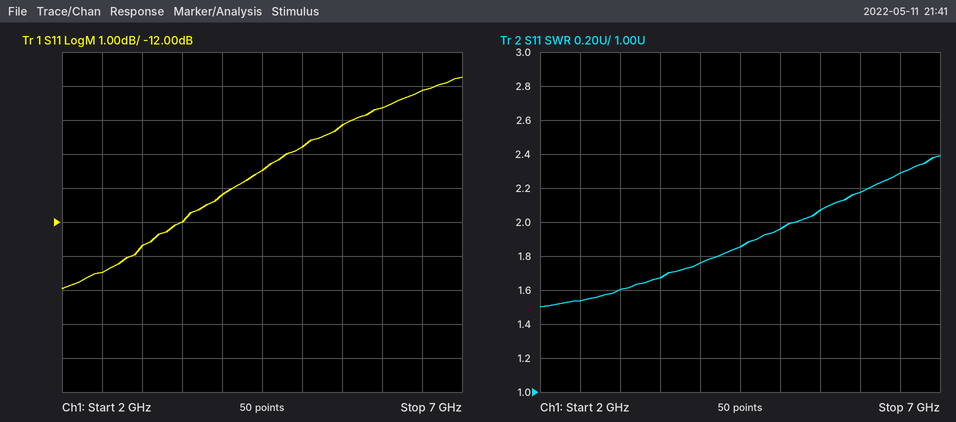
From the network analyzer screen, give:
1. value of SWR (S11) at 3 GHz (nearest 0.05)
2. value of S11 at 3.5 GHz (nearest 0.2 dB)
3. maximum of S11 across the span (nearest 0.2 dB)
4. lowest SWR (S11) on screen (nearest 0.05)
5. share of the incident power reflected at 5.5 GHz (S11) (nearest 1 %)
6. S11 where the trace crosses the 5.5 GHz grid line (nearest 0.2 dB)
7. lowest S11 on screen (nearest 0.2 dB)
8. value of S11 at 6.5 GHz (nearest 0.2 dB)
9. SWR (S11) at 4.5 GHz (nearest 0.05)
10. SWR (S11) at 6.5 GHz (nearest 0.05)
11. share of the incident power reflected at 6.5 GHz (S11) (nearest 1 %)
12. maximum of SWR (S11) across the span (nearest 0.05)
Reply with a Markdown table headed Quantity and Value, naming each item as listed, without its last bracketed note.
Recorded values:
| Quantity | Value |
|---|---|
| value of SWR (S11) at 3 GHz | 1.60 |
| value of S11 at 3.5 GHz | -12.0 dB |
| maximum of S11 across the span | -7.8 dB |
| lowest SWR (S11) on screen | 1.50 |
| share of the incident power reflected at 5.5 GHz (S11) | 12 % |
| S11 where the trace crosses the 5.5 GHz grid line | -9.2 dB |
| lowest S11 on screen | -14.0 dB |
| value of S11 at 6.5 GHz | -8.2 dB |
| SWR (S11) at 4.5 GHz | 1.85 |
| SWR (S11) at 6.5 GHz | 2.30 |
| share of the incident power reflected at 6.5 GHz (S11) | 15 % |
| maximum of SWR (S11) across the span | 2.40 |
